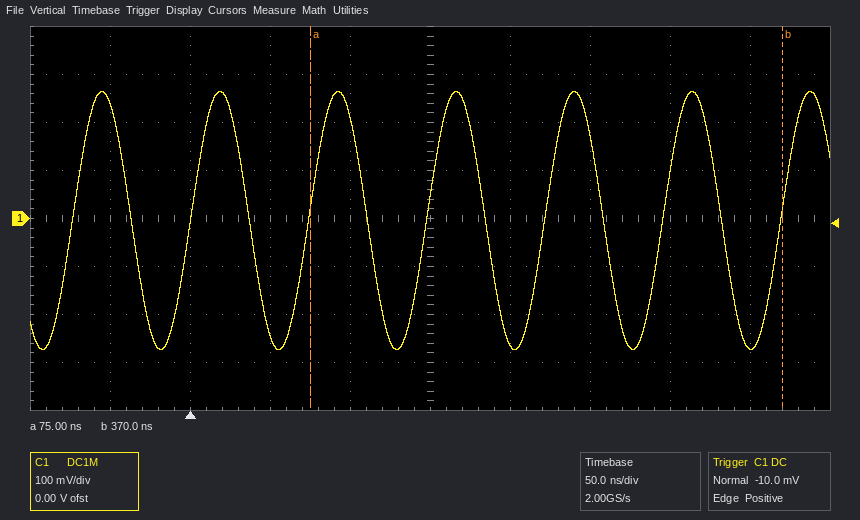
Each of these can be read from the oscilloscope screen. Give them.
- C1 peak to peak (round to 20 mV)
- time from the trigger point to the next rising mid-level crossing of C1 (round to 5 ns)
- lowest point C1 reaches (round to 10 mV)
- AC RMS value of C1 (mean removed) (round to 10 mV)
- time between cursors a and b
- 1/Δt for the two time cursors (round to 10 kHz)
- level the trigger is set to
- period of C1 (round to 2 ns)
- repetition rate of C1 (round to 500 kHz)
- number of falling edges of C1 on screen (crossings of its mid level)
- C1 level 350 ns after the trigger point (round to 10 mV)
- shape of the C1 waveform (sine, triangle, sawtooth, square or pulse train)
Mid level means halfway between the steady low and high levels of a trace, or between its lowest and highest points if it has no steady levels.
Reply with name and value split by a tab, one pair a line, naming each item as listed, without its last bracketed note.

C1 peak to peak	540 mV
time from the trigger point to the next rising mid-level crossing of C1	75 ns
lowest point C1 reaches	-270 mV
AC RMS value of C1 (mean removed)	190 mV
time between cursors a and b	295 ns
1/Δt for the two time cursors	3.39 MHz
level the trigger is set to	-10.0 mV
period of C1	74 ns
repetition rate of C1	13.5 MHz
number of falling edges of C1 on screen	6
C1 level 350 ns after the trigger point	-270 mV
shape of the C1 waveform	sine
